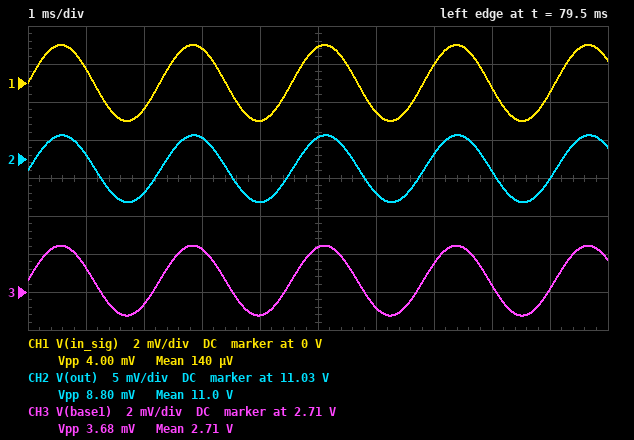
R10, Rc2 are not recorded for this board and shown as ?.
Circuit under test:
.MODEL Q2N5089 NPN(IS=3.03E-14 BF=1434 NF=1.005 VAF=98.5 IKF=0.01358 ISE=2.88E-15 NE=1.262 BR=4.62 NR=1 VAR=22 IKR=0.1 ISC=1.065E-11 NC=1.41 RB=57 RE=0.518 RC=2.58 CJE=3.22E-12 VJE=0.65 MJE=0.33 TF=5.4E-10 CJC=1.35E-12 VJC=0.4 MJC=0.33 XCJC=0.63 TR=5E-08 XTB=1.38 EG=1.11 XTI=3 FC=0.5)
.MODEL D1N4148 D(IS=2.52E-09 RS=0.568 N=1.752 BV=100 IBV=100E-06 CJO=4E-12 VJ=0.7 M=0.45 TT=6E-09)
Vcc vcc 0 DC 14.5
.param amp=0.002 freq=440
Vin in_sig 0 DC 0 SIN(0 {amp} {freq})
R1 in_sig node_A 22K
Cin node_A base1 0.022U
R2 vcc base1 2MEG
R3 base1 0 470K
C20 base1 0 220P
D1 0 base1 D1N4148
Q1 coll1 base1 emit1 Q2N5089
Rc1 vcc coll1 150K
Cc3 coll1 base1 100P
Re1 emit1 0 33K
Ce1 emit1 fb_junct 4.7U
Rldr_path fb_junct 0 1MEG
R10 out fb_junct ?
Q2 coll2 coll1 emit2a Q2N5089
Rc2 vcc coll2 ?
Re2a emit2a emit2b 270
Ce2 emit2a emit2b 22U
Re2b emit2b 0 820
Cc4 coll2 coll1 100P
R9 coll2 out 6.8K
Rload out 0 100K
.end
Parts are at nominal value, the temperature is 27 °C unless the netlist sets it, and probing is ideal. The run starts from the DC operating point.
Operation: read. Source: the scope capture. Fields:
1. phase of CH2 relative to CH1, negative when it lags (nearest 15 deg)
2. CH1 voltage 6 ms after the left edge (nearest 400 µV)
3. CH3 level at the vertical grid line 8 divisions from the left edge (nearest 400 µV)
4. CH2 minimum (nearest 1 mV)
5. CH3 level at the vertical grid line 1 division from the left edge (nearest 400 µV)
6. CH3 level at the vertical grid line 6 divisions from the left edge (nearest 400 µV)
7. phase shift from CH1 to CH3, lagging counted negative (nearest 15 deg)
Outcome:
0 deg
-1.6 mV
2.7104 V
11.024 V
2.7112 V
2.7092 V
0 deg
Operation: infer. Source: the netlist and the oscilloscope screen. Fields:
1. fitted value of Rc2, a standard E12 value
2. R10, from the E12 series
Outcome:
820 Ω
180 kΩ
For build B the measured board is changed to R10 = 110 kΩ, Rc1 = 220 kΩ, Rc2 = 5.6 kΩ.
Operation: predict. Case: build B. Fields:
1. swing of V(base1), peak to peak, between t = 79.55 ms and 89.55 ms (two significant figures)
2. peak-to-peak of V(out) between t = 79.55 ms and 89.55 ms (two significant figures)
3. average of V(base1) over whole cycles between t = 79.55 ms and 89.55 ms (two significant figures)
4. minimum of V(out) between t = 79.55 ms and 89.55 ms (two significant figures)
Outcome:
2.3 mV
2.7 mV
2.4 V
6.6 V
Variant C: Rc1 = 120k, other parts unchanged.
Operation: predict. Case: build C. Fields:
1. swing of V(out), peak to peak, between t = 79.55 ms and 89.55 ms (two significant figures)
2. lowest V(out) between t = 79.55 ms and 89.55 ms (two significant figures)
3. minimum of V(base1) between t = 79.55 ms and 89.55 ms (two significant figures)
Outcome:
7.7 mV
9.8 V
2.7 V
